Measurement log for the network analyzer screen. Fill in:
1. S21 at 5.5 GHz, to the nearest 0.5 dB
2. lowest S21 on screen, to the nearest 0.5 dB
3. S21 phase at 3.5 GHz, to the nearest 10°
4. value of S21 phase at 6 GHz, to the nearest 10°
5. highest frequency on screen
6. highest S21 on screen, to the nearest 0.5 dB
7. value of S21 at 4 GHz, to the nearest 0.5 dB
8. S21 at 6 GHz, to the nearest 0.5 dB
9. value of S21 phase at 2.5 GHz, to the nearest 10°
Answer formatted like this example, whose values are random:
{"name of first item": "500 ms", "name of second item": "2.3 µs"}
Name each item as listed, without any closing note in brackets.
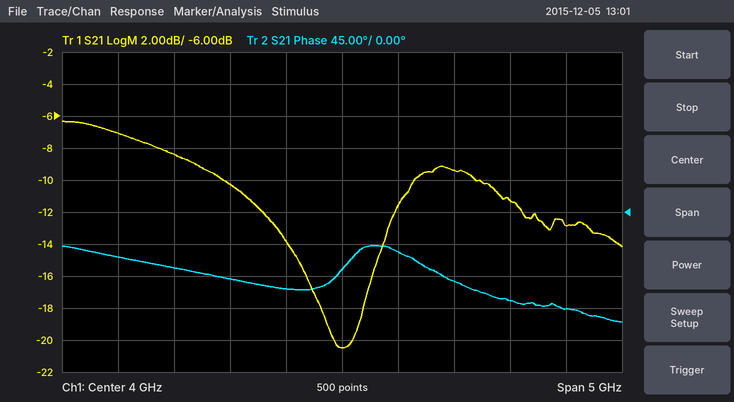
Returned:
{"S21 at 5.5 GHz, to the nearest 0.5 dB": "-11.5 dB", "lowest S21 on screen, to the nearest 0.5 dB": "-20.5 dB", "S21 phase at 3.5 GHz, to the nearest 10°": "-110°", "value of S21 phase at 6 GHz, to the nearest 10°": "-140°", "highest frequency on screen": "6.5 GHz", "highest S21 on screen, to the nearest 0.5 dB": "-6.5 dB", "value of S21 at 4 GHz, to the nearest 0.5 dB": "-20.5 dB", "S21 at 6 GHz, to the nearest 0.5 dB": "-13.0 dB", "value of S21 phase at 2.5 GHz, to the nearest 10°": "-80°"}
